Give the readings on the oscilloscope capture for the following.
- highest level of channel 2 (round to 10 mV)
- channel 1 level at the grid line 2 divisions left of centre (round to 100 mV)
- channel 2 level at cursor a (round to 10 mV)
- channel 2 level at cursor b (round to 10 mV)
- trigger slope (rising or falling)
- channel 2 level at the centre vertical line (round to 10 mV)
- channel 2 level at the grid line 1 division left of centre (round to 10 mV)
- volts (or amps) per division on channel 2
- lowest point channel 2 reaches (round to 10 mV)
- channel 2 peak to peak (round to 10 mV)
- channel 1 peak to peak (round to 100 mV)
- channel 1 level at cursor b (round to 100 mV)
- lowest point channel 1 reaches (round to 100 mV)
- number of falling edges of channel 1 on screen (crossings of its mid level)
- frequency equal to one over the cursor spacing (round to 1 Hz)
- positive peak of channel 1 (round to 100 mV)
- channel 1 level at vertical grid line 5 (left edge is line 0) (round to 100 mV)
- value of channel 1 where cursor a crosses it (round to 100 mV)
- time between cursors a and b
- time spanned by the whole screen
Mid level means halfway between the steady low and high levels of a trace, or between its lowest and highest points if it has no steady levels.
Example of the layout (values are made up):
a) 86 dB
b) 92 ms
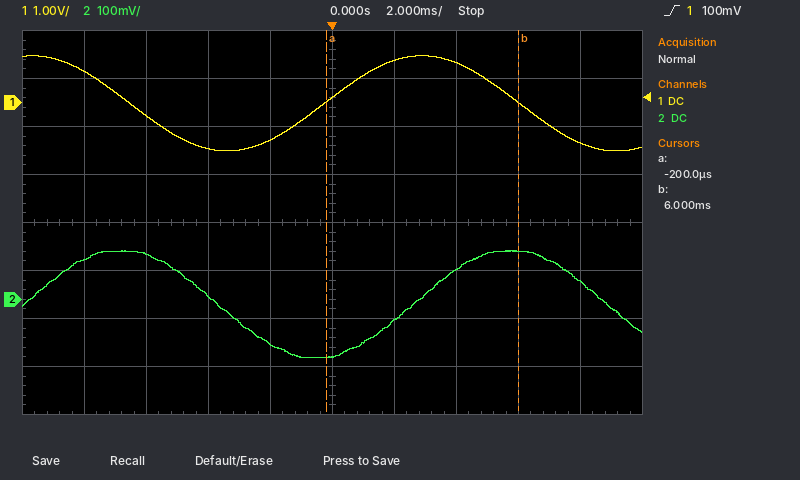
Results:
a) 100 mV
b) -1.0 V
c) -120 mV
d) 100 mV
e) rising
f) -120 mV
g) -90 mV
h) 100 mV
i) -120 mV
j) 220 mV
k) 2.0 V
l) 0.0 V
m) -1.0 V
n) 2
o) 161 Hz
p) 1.0 V
q) 100 mV
r) 0.0 V
s) 6.2 ms
t) 20 ms
